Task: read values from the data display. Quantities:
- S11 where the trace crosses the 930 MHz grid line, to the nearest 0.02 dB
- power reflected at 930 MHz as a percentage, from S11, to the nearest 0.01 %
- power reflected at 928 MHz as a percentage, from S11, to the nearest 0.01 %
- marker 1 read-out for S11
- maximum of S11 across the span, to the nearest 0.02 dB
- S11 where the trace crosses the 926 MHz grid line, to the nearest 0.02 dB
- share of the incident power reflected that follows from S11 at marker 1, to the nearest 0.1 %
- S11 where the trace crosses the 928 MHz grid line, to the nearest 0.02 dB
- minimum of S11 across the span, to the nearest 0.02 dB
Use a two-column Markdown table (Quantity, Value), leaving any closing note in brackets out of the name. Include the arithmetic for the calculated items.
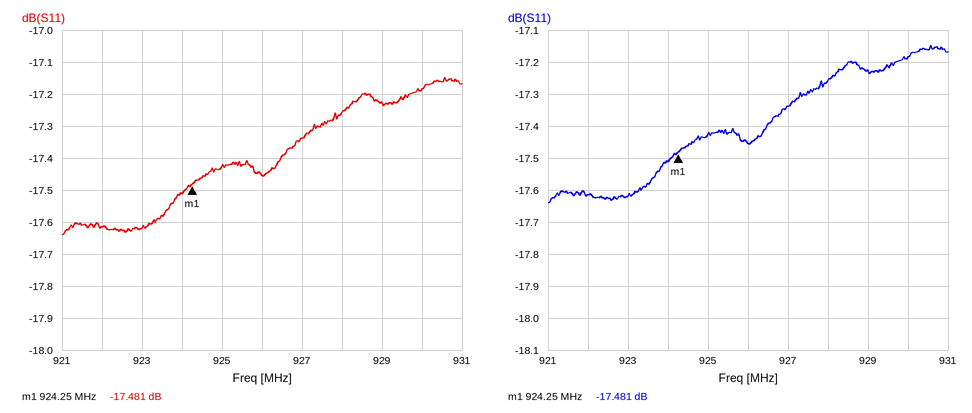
| Quantity | Value |
|---|---|
| S11 where the trace crosses the 930 MHz grid line, to the nearest 0.02 dB | -17.18 dB |
| power reflected at 930 MHz as a percentage, from S11, to the nearest 0.01 % | 10^(-17.18/10) ≈ 1.91 % |
| power reflected at 928 MHz as a percentage, from S11, to the nearest 0.01 % | 10^(-17.26/10) ≈ 1.88 % |
| marker 1 read-out for S11 | -17.481 dB |
| maximum of S11 across the span, to the nearest 0.02 dB | -17.14 dB |
| S11 where the trace crosses the 926 MHz grid line, to the nearest 0.02 dB | -17.46 dB |
| share of the incident power reflected that follows from S11 at marker 1, to the nearest 0.1 % | 10^(-17.481/10) ≈ 1.8 % |
| S11 where the trace crosses the 928 MHz grid line, to the nearest 0.02 dB | -17.26 dB |
| minimum of S11 across the span, to the nearest 0.02 dB | -17.64 dB |
